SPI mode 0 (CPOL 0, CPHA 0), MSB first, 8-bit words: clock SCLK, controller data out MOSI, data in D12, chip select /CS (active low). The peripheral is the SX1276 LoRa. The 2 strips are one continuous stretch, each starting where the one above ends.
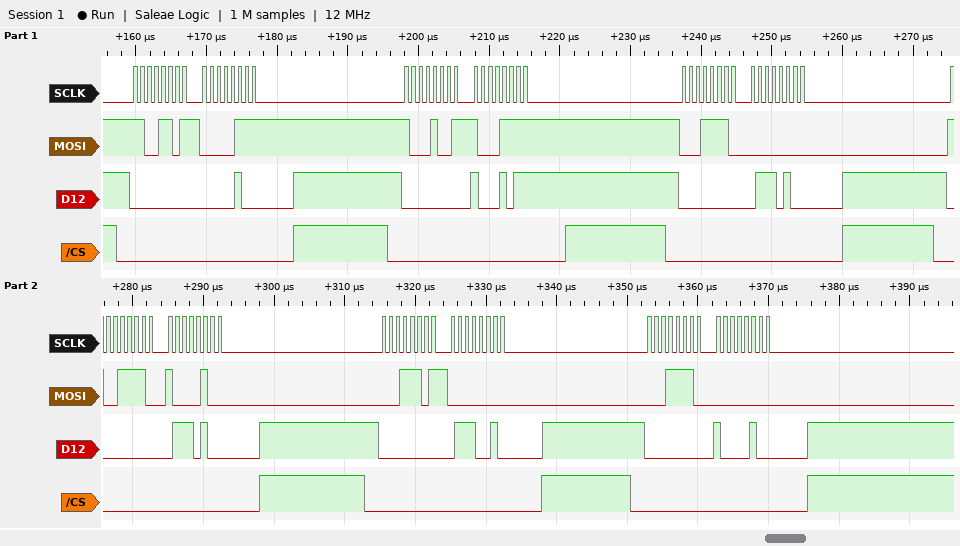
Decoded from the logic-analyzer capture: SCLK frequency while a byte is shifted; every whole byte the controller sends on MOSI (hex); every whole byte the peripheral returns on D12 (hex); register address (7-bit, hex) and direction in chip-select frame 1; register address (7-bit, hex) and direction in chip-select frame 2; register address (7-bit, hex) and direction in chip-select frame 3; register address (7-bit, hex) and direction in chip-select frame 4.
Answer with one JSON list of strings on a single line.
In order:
["1 MHz", "CD 07 89 8F 1E 00 9E 84 1D 00 1E 00", "00 04 00 8B 00 74 00 74 00 72 00 84", "0x4D write", "0x09 write", "0x1E read", "0x1E write"]
